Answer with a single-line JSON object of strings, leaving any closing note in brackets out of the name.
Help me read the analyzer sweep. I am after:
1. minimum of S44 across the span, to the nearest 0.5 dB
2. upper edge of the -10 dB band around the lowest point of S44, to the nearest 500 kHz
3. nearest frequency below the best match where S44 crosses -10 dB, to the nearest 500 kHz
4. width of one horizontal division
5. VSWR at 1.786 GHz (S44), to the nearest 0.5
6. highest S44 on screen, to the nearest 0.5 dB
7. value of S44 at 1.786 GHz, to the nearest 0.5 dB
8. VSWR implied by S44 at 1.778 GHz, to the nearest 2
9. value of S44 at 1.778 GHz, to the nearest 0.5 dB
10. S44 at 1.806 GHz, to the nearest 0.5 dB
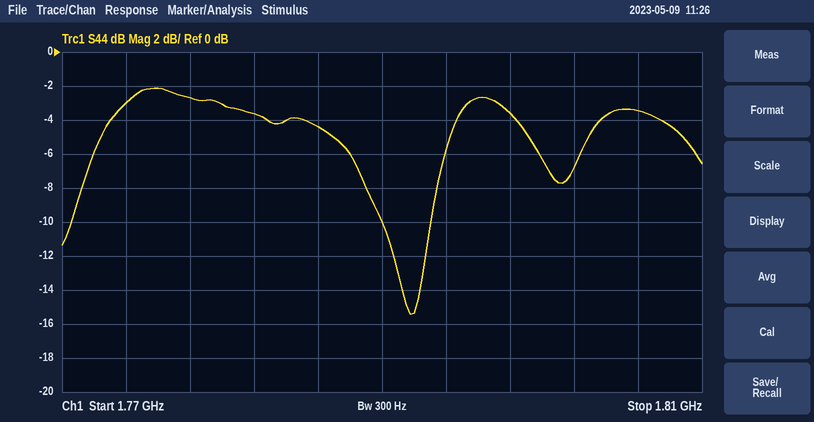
{"minimum of S44 across the span, to the nearest 0.5 dB": "-15.5 dB", "upper edge of the -10 dB band around the lowest point of S44, to the nearest 500 kHz": "1.7930 GHz", "nearest frequency below the best match where S44 crosses -10 dB, to the nearest 500 kHz": "1.7900 GHz", "width of one horizontal division": "4 MHz", "VSWR at 1.786 GHz (S44), to the nearest 0.5": "4.0", "highest S44 on screen, to the nearest 0.5 dB": "-2.0 dB", "value of S44 at 1.786 GHz, to the nearest 0.5 dB": "-4.5 dB", "VSWR implied by S44 at 1.778 GHz, to the nearest 2": "6", "value of S44 at 1.778 GHz, to the nearest 0.5 dB": "-2.5 dB", "S44 at 1.806 GHz, to the nearest 0.5 dB": "-3.5 dB"}
